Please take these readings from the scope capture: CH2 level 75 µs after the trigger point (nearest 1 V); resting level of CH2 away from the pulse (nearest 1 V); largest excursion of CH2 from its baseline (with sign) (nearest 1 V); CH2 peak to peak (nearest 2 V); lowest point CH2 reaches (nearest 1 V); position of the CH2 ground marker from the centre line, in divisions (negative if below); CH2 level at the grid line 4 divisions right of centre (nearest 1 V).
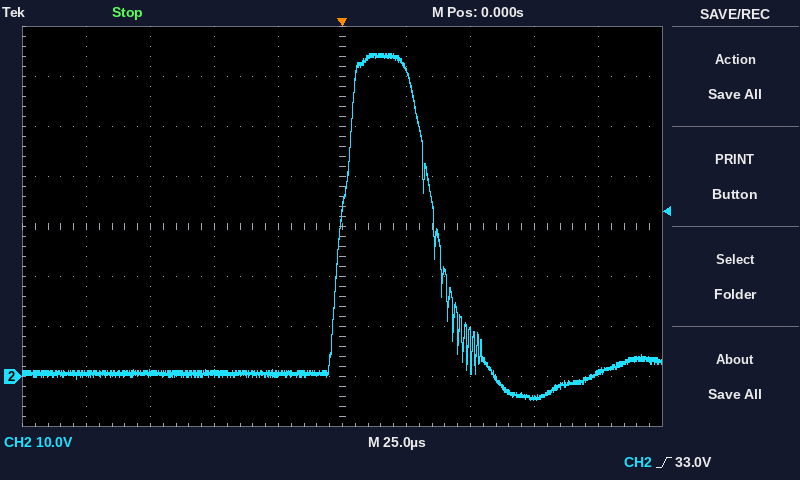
-4 V
1 V
+64 V
70 V
-5 V
-3.0 div
1 V
